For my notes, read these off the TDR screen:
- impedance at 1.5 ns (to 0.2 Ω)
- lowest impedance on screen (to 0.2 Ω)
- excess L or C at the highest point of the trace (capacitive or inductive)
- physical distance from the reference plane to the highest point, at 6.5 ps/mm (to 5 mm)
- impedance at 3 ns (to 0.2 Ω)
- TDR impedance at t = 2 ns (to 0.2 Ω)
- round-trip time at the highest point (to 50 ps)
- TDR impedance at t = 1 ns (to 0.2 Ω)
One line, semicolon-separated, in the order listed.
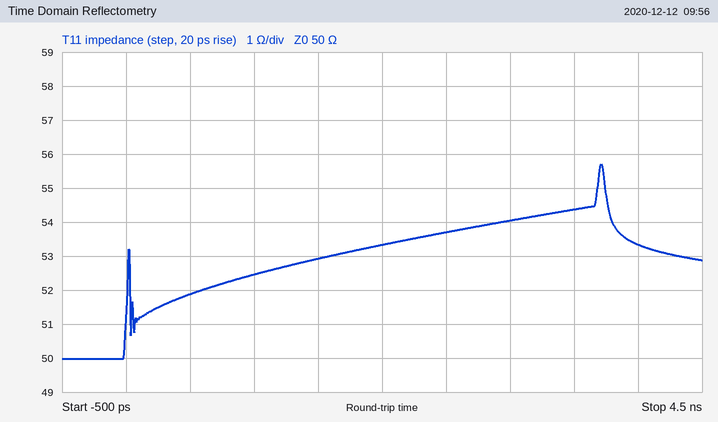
53.0 Ω; 50.0 Ω; inductive; 285 mm; 54.0 Ω; 53.4 Ω; 3.70 ns; 52.4 Ω
